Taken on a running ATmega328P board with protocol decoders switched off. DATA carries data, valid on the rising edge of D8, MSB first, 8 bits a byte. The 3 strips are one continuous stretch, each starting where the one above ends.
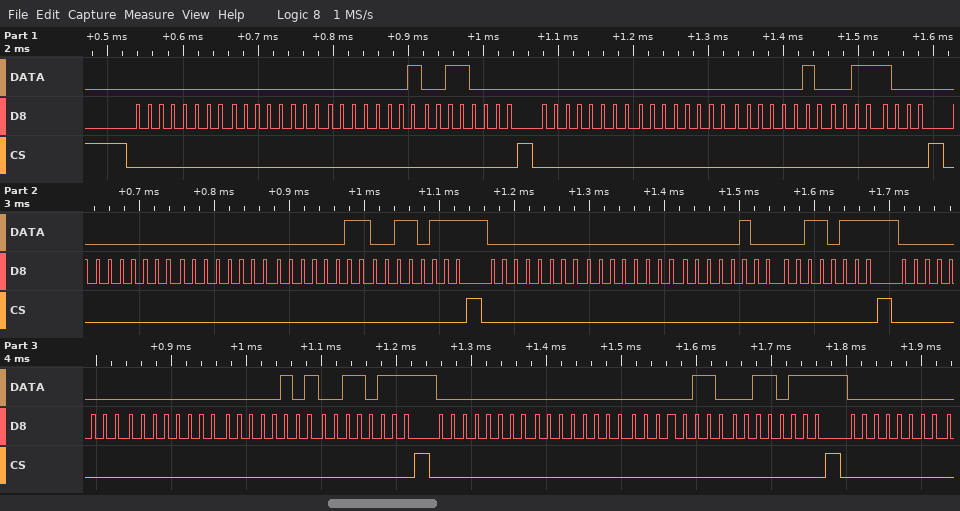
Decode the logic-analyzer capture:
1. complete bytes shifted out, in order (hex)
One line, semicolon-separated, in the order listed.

00 00 01 30 00 00 02 38 00 00 03 37 00 00 04 37 00 00 05 37 00 00 06 37 00
